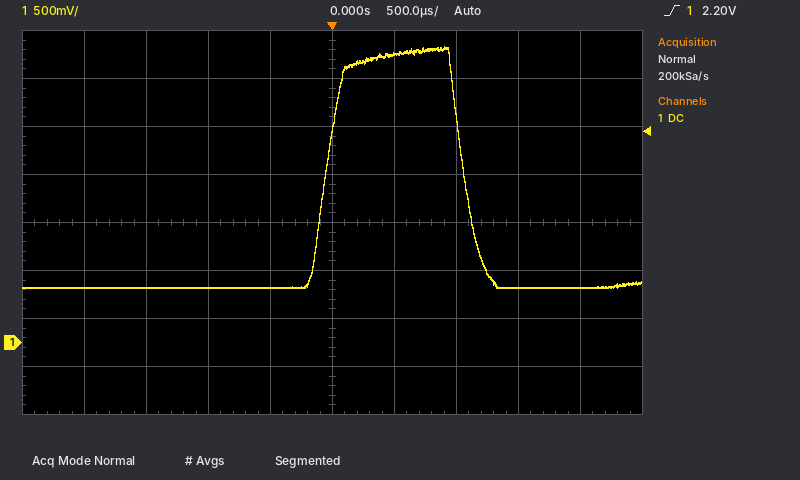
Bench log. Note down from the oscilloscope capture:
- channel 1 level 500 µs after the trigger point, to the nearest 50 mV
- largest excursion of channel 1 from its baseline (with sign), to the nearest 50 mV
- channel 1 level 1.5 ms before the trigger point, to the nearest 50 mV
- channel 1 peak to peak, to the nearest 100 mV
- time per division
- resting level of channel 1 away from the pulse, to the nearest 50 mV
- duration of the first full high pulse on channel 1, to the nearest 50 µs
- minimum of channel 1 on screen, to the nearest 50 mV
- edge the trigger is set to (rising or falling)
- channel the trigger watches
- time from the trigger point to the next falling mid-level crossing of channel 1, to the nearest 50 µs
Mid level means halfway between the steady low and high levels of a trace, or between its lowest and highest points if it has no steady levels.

3.00 V
+2.50 V
550 mV
2.50 V
500 µs
550 mV
1.10 ms
550 mV
rising
channel 1
1.05 ms
